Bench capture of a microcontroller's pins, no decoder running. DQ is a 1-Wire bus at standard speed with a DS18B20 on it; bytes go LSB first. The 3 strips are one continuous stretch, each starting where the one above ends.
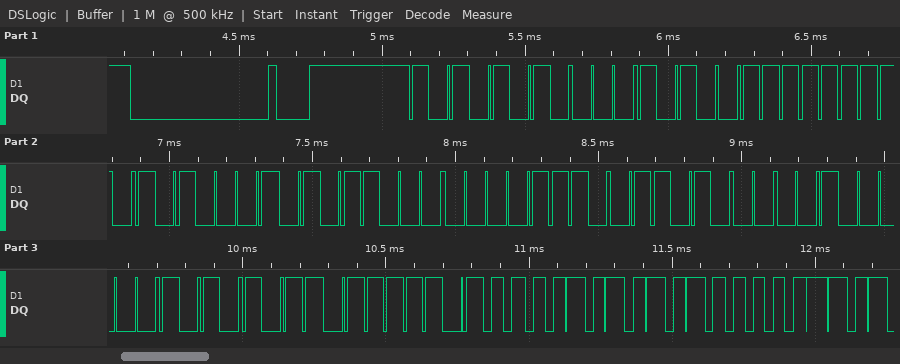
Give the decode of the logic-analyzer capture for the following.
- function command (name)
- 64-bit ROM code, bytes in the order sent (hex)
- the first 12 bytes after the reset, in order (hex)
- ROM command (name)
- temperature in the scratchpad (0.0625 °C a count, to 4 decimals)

Read Scratchpad
28 FF 8A 1A 70 16 04 D5
55 28 FF 8A 1A 70 16 04 D5 BE 50 05
Match ROM
85.0000 °C
